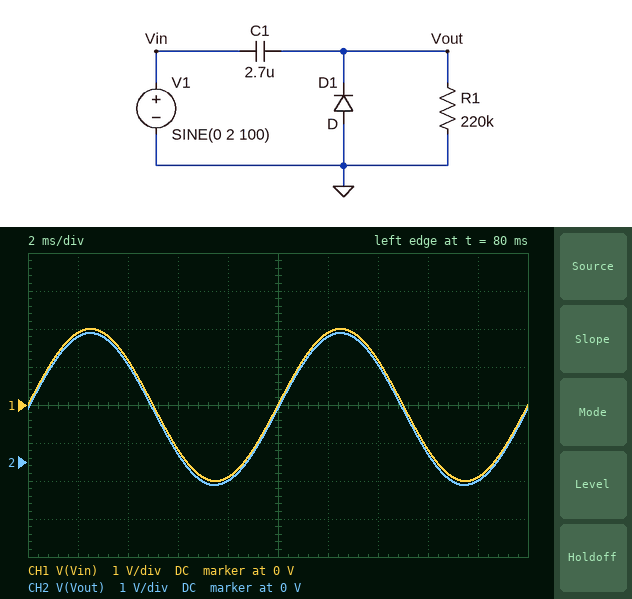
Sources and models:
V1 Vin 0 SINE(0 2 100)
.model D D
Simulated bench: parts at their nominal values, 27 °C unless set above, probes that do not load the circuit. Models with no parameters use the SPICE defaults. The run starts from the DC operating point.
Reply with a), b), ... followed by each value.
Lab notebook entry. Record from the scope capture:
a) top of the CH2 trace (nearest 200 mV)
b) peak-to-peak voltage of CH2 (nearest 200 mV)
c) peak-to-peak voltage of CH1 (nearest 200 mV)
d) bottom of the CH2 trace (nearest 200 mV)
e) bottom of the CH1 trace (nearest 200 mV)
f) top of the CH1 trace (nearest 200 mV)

a) 3.4 V
b) 4.0 V
c) 4.0 V
d) -600 mV
e) -2.0 V
f) 2.0 V
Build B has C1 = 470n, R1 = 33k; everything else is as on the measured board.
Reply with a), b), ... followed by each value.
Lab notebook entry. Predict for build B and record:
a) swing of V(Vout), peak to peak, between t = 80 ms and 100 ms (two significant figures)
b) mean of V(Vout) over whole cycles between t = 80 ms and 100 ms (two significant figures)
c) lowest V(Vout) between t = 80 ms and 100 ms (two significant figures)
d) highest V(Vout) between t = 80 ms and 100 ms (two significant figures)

a) 3.7 V
b) 1.1 V
c) -630 mV
d) 3.0 V
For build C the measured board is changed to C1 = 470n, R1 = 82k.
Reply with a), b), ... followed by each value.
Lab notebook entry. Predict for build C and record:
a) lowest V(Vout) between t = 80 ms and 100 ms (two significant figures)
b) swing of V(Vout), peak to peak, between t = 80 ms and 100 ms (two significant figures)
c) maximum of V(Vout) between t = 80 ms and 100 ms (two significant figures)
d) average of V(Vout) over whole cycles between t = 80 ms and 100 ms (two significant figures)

a) -620 mV
b) 3.9 V
c) 3.3 V
d) 1.3 V
